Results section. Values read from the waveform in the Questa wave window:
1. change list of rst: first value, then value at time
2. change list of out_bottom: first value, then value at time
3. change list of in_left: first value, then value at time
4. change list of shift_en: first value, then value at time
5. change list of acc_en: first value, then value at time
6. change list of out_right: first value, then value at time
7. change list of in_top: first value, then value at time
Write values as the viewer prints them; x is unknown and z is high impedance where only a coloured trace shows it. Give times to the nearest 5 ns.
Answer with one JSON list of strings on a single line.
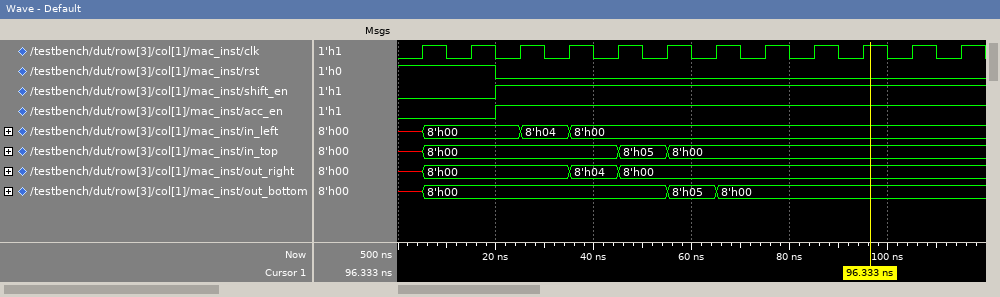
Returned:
["1, 0 at 20 ns", "x, 8'h00 at 5 ns, 8'h05 at 55 ns, 8'h00 at 65 ns", "x, 8'h00 at 5 ns, 8'h04 at 25 ns, 8'h00 at 35 ns", "0, 1 at 20 ns", "0, 1 at 20 ns", "x, 8'h00 at 5 ns, 8'h04 at 35 ns, 8'h00 at 45 ns", "x, 8'h00 at 5 ns, 8'h05 at 45 ns, 8'h00 at 55 ns"]
